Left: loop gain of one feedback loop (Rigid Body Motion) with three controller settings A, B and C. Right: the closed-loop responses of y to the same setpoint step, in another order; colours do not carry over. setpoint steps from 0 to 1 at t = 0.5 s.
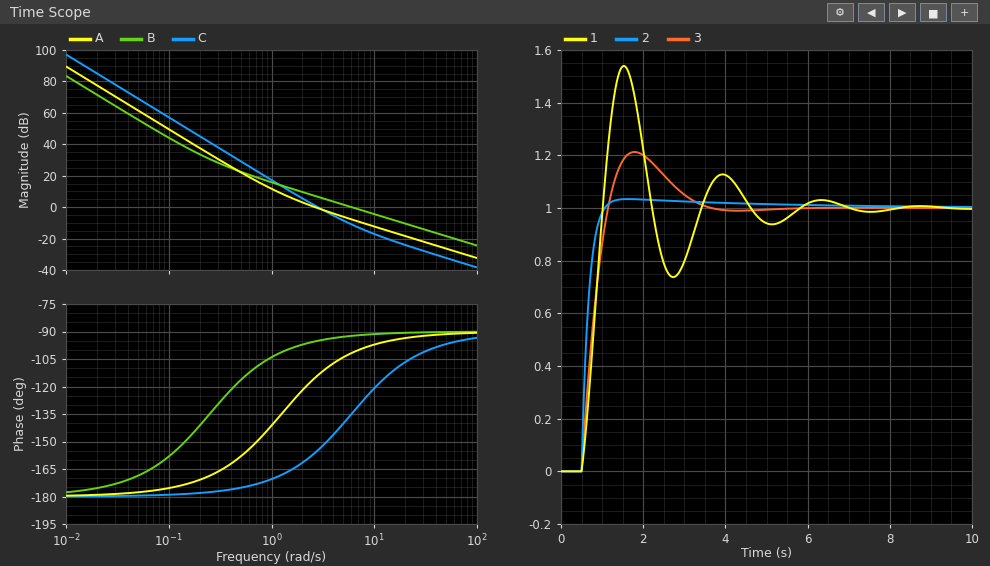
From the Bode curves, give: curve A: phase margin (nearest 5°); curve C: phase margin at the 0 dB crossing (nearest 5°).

65°
25°
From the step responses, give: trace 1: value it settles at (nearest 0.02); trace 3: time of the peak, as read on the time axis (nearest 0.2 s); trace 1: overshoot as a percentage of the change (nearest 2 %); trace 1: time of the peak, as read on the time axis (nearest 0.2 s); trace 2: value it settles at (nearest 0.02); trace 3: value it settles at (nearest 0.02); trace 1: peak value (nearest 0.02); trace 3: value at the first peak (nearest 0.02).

1.00
1.8 s
54 %
1.6 s
1.00
1.00
1.54
1.22
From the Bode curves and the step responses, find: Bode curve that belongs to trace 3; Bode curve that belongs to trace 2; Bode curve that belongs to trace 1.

A
B
C
